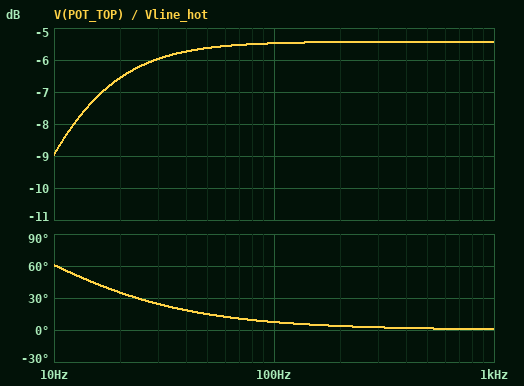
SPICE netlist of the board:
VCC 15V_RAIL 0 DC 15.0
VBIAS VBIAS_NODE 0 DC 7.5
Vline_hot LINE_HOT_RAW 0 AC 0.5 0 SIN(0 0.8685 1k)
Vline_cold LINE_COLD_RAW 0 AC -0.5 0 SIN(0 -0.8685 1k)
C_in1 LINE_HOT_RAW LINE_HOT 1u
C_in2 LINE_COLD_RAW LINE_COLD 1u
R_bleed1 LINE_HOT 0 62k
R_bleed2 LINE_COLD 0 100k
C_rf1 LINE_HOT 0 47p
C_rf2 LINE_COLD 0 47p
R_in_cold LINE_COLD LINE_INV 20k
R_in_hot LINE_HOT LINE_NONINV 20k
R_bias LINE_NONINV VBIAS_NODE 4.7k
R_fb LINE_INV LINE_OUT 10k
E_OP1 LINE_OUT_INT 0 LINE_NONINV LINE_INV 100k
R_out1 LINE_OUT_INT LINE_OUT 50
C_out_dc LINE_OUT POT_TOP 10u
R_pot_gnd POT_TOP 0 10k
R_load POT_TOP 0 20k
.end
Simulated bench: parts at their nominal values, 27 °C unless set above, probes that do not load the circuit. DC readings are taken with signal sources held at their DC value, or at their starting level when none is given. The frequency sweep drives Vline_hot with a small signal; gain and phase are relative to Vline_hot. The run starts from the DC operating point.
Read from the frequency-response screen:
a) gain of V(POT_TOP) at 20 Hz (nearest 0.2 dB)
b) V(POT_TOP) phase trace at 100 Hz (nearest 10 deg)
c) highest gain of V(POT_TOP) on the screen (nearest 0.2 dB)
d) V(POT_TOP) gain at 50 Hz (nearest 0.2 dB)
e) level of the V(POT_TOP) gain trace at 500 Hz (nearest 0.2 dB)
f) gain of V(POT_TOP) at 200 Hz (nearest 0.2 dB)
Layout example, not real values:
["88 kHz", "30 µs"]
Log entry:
["-6.6 dB", "10 deg", "-5.4 dB", "-5.6 dB", "-5.4 dB", "-5.4 dB"]
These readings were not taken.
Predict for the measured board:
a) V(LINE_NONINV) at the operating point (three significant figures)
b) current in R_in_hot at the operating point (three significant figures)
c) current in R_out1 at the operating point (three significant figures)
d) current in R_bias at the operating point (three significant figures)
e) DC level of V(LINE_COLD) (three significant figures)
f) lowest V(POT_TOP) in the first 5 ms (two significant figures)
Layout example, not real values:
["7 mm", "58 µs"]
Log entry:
["7.09 V", "86.5 µA", "59.1 µA", "86.5 µA", "5.91 V", "-690 mV"]
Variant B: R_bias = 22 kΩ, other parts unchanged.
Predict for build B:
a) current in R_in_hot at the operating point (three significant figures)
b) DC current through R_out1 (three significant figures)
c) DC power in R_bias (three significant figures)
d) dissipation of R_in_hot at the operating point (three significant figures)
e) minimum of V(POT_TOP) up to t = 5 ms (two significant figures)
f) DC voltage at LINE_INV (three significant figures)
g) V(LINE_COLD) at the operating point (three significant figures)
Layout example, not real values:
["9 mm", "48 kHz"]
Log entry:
["72.1 µA", "49.3 µA", "114 µW", "104 µW", "-1.1 V", "5.91 V", "4.93 V"]
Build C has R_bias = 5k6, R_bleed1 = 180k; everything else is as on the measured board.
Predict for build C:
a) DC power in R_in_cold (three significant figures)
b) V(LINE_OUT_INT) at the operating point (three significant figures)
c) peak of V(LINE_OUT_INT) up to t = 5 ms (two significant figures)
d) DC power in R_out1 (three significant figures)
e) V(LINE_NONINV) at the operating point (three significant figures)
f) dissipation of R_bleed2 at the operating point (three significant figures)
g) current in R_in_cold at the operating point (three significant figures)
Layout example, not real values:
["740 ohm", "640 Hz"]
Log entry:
["73.9 µW", "7.91 V", "8.6 V", "185 nW", "7.30 V", "370 µW", "60.8 µA"]
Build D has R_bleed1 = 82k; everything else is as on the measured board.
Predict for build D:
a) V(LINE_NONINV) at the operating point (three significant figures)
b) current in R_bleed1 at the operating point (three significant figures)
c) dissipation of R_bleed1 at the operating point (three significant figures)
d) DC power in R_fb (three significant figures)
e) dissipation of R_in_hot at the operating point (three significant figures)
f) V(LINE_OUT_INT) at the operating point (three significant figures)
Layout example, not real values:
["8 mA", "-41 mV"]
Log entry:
["7.17 V", "70.3 µA", "405 µW", "35.7 µW", "98.8 µW", "7.77 V"]
